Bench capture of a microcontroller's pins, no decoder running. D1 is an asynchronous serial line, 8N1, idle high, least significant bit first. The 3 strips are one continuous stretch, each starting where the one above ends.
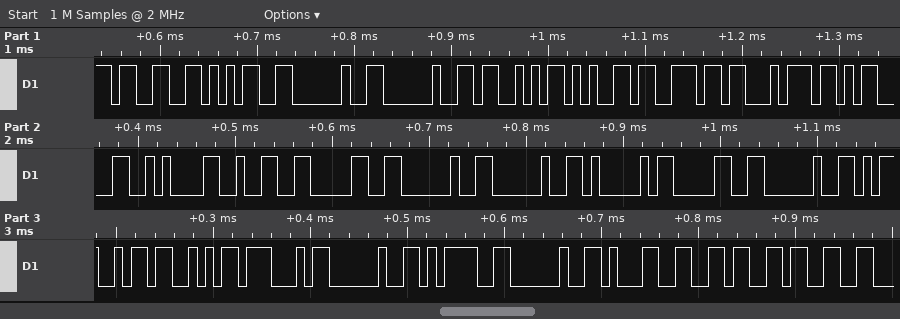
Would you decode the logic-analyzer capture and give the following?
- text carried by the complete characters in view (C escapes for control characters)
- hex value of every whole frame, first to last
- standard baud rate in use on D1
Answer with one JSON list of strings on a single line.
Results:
["\"35  Sent\\r\\n20  A0 MSG = 163\"", "33 35 20 20 53 65 6E 74 0D 0A 32 30 20 20 41 30 20 4D 53 47 20 3D 20 31 36 33", "115200 baud"]
